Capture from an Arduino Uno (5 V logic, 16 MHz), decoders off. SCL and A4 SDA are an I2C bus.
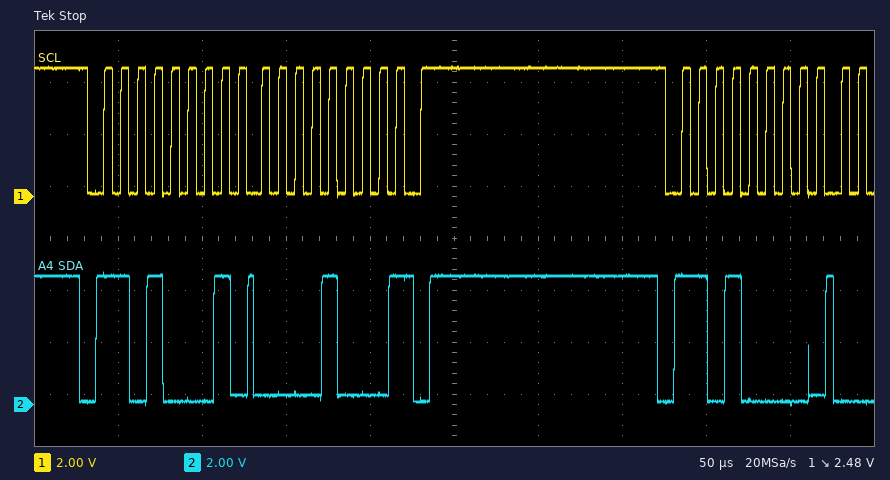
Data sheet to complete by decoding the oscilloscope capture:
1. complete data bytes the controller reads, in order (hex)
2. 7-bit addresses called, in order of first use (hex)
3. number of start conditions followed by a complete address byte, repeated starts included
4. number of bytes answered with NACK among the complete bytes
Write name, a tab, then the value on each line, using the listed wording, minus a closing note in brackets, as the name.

complete data bytes the controller reads, in order	08
7-bit addresses called, in order of first use	0x68
number of start conditions followed by a complete address byte, repeated starts included	2
number of bytes answered with NACK among the complete bytes	1
